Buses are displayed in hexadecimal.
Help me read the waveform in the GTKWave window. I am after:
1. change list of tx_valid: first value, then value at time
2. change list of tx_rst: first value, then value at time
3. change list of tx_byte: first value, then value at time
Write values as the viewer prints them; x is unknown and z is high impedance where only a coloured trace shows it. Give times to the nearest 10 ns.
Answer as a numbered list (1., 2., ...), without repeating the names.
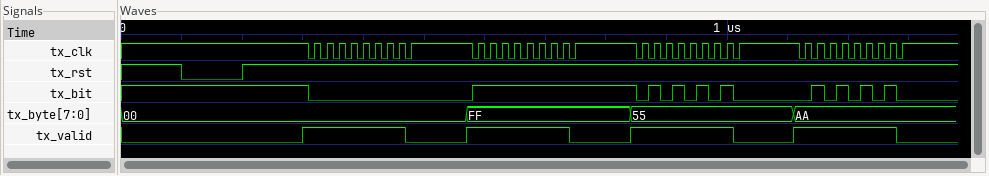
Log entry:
1. 0, 1 at 300 ns, 0 at 470 ns, 1 at 570 ns, 0 at 740 ns, 1 at 840 ns, 0 at 1010 ns, 1 at 1110 ns, 0 at 1280 ns
2. 1, 0 at 100 ns, 1 at 200 ns
3. 00, FF at 570 ns, 55 at 840 ns, AA at 1110 ns
